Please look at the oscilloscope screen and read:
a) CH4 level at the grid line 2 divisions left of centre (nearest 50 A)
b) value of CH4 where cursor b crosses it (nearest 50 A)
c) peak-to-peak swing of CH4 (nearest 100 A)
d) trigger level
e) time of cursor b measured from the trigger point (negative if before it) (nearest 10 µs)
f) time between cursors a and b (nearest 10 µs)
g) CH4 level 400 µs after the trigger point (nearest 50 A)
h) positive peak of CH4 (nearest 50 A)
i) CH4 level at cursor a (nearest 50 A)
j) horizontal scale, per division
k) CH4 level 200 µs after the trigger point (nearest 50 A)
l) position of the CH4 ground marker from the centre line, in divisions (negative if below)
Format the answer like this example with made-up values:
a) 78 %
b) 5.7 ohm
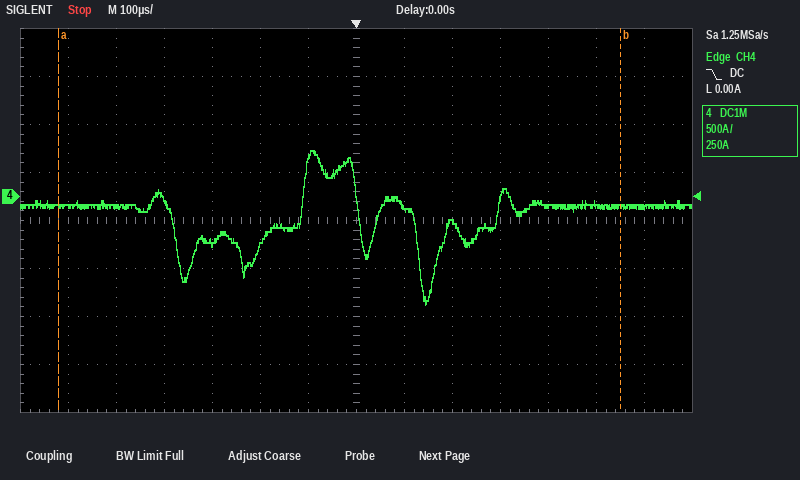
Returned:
a) -500 A
b) -100 A
c) 1.60 kA
d) 0.00 A
e) +550 µs
f) 1.17 ms
g) -100 A
h) 500 A
i) -100 A
j) 100 µs
k) -250 A
l) +0.5 div
